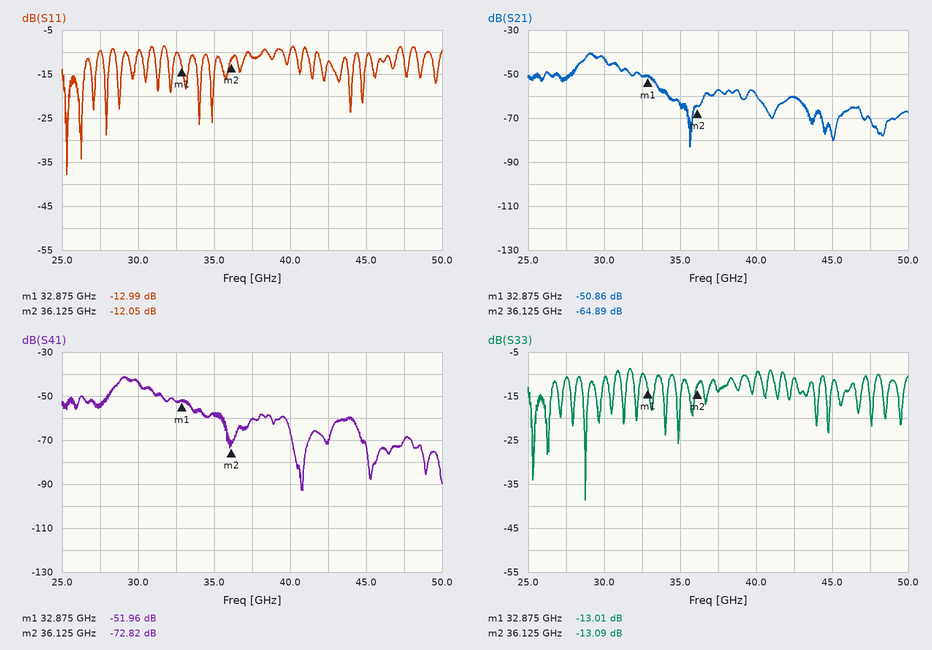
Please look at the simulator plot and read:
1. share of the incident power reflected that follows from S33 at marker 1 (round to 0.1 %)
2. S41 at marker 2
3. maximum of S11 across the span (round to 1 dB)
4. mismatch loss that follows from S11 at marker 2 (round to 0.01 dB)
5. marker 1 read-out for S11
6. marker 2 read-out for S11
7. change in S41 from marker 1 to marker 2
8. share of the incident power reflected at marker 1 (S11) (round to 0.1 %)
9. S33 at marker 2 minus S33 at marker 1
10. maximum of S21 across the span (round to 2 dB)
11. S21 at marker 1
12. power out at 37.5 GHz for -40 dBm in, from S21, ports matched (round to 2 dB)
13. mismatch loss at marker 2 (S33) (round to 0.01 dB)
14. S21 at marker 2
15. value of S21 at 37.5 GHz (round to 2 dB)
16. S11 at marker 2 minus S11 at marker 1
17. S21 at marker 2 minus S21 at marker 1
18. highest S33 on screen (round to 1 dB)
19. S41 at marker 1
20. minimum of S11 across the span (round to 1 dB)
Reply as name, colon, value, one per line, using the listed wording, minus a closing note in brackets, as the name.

share of the incident power reflected that follows from S33 at marker 1: 5.0 %
S41 at marker 2: -72.82 dB
maximum of S11 across the span: -9 dB
mismatch loss that follows from S11 at marker 2: 0.28 dB
marker 1 read-out for S11: -12.99 dB
marker 2 read-out for S11: -12.05 dB
change in S41 from marker 1 to marker 2: -20.86 dB
share of the incident power reflected at marker 1 (S11): 5.0 %
S33 at marker 2 minus S33 at marker 1: -0.08 dB
maximum of S21 across the span: -40 dB
S21 at marker 1: -50.86 dB
power out at 37.5 GHz for -40 dBm in, from S21, ports matched: -98 dBm
mismatch loss at marker 2 (S33): 0.22 dB
S21 at marker 2: -64.89 dB
value of S21 at 37.5 GHz: -58 dB
S11 at marker 2 minus S11 at marker 1: 0.94 dB
S21 at marker 2 minus S21 at marker 1: -14.03 dB
highest S33 on screen: -9 dB
S41 at marker 1: -51.96 dB
minimum of S11 across the span: -38 dB
